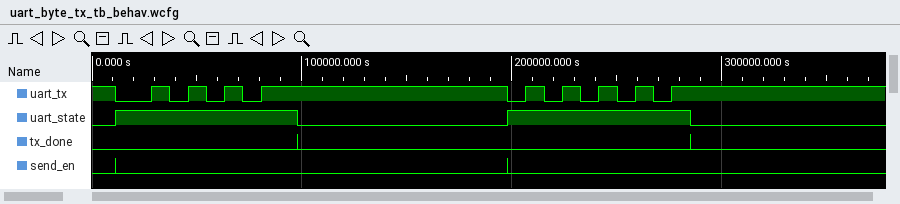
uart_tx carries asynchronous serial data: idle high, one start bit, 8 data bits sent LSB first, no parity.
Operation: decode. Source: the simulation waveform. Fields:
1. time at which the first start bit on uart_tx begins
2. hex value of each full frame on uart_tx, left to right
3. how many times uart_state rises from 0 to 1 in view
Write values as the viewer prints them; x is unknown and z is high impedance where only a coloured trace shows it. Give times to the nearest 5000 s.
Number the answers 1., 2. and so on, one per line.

1. 10000 s
2. AA, 55
3. 2
